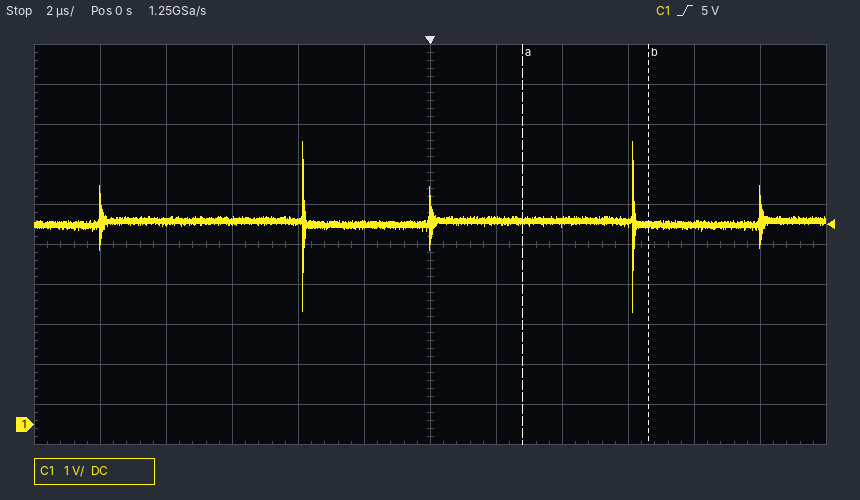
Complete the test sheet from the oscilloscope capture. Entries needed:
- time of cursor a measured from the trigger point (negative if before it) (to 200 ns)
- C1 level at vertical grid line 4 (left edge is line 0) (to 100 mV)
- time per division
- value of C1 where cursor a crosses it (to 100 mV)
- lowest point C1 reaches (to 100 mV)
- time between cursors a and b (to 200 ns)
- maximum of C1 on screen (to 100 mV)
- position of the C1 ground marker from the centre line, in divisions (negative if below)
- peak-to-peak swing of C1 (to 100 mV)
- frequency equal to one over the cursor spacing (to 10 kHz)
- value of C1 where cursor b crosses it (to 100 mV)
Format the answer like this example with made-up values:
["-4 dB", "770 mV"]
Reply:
["+2.8 µs", "5.1 V", "2 µs", "5.1 V", "2.8 V", "3.8 µs", "7.1 V", "-4.5 div", "4.3 V", "260 kHz", "5.0 V"]
